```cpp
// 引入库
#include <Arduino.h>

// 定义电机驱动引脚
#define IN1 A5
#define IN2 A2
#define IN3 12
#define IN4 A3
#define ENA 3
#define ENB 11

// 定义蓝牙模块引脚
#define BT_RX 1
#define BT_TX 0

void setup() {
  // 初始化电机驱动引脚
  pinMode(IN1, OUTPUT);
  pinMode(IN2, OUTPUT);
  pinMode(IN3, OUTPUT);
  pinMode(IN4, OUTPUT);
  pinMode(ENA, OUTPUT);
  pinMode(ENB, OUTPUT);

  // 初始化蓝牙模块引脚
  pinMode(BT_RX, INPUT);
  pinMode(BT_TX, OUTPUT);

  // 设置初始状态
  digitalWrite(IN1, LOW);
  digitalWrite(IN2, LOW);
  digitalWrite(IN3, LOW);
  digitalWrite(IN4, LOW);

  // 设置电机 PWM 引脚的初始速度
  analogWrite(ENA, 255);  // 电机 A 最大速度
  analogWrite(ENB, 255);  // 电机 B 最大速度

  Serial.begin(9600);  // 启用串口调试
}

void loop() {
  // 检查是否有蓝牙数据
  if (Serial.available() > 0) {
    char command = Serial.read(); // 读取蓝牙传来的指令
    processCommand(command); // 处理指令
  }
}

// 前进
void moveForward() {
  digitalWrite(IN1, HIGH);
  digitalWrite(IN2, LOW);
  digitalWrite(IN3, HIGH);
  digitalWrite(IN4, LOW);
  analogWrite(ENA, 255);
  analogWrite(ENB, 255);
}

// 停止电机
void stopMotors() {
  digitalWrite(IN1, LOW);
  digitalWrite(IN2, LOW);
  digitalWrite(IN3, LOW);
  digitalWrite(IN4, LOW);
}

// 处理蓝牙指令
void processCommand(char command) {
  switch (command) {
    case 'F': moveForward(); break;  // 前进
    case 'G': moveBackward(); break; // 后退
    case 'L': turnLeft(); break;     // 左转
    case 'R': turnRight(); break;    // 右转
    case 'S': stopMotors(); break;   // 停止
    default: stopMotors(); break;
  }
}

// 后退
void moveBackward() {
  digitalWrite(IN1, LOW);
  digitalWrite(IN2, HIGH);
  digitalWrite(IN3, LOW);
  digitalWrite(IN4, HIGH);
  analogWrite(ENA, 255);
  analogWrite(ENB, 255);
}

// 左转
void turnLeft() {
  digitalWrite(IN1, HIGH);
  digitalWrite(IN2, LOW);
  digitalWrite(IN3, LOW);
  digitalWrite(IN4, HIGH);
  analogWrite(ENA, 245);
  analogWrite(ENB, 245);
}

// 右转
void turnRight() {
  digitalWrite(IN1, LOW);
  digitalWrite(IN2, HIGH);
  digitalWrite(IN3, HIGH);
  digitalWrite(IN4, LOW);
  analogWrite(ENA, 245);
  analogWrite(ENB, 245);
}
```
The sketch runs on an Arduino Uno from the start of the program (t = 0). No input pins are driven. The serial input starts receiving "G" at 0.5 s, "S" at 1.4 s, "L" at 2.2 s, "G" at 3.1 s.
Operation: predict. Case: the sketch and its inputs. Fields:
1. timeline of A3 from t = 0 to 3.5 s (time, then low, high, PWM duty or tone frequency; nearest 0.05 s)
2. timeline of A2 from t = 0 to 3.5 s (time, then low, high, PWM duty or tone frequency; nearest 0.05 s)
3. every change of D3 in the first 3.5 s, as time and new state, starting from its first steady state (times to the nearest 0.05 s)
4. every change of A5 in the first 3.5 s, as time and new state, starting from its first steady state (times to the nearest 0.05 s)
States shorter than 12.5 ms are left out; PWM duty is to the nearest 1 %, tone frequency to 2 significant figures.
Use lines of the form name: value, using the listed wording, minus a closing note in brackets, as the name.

timeline of A3 from t = 0 to 3.5 s: 0 s low; 0.5 s high; 1.4 s low; 2.2 s high
timeline of A2 from t = 0 to 3.5 s: 0 s low; 0.5 s high; 1.4 s low; 3.1 s high
every change of D3 in the first 3.5 s, as time and new state, starting from its first steady state: 0 s high; 2.2 s PWM 96 %; 3.1 s high
every change of A5 in the first 3.5 s, as time and new state, starting from its first steady state: 0 s low; 2.2 s high; 3.1 s low
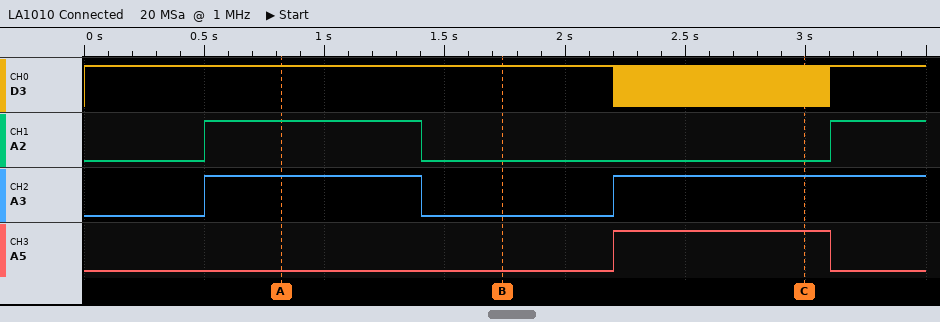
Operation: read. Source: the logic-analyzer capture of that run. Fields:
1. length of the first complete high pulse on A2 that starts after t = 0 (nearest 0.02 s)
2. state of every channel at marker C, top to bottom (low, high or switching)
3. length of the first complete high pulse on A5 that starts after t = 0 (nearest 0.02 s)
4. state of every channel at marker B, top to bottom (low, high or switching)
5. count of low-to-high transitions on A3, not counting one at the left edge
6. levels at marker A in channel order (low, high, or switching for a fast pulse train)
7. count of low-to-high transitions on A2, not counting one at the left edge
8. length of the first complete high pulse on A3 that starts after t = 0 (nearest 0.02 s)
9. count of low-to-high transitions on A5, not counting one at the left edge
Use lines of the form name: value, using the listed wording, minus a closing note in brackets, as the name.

length of the first complete high pulse on A2 that starts after t = 0: 0.90 s
state of every channel at marker C, top to bottom: D3 switching, A2 low, A3 high, A5 high
length of the first complete high pulse on A5 that starts after t = 0: 0.90 s
state of every channel at marker B, top to bottom: D3 high, A2 low, A3 low, A5 low
count of low-to-high transitions on A3, not counting one at the left edge: 2
levels at marker A in channel order: D3 high, A2 high, A3 high, A5 low
count of low-to-high transitions on A2, not counting one at the left edge: 2
length of the first complete high pulse on A3 that starts after t = 0: 0.90 s
count of low-to-high transitions on A5, not counting one at the left edge: 1
